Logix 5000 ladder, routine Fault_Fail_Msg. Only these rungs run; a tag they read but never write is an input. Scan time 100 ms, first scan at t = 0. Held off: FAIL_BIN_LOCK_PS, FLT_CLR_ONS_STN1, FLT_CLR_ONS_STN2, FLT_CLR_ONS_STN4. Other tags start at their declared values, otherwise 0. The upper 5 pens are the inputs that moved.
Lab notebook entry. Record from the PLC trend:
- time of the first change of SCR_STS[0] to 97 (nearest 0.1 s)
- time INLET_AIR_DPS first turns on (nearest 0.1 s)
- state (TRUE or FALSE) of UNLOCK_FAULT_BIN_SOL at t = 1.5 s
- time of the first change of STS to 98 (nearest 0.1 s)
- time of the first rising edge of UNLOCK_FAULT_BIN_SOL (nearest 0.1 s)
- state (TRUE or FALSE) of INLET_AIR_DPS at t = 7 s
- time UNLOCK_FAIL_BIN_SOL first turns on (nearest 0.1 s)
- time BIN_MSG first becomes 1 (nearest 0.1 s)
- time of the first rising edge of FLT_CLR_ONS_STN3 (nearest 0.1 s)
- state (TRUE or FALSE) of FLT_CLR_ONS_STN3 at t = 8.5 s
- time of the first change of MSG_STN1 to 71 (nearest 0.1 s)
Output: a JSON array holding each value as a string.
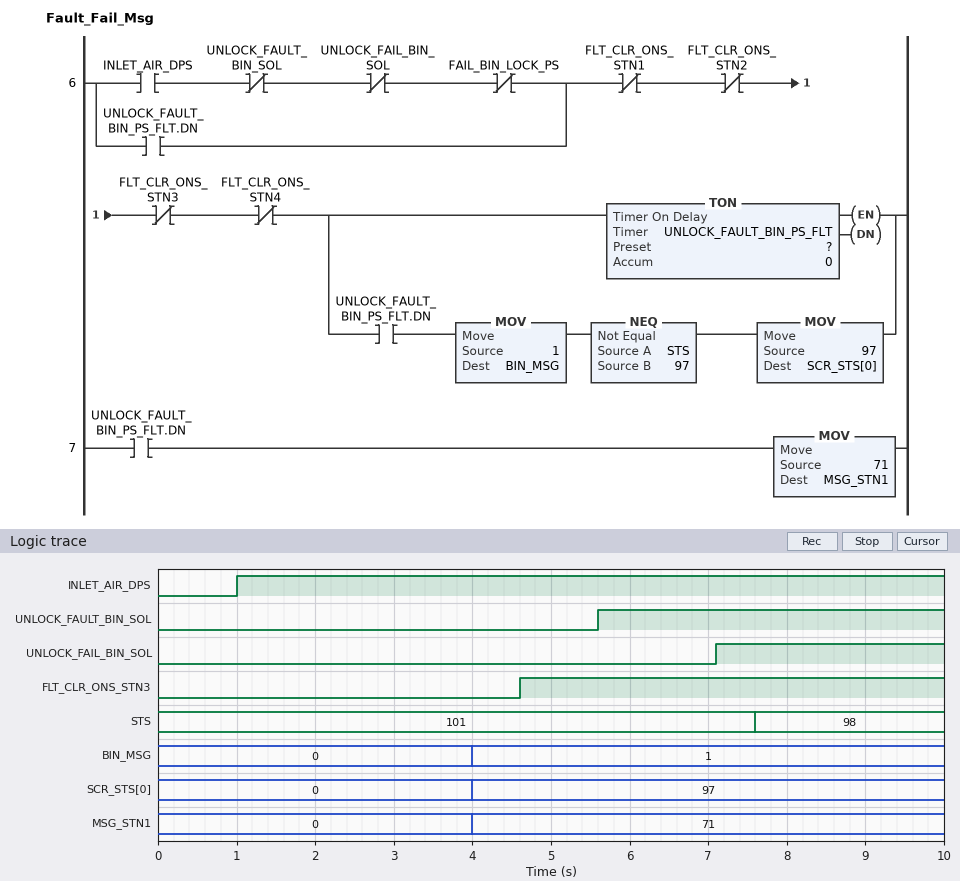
["4.0 s", "1.0 s", "FALSE", "7.6 s", "5.6 s", "TRUE", "7.1 s", "4.0 s", "4.6 s", "TRUE", "4.0 s"]
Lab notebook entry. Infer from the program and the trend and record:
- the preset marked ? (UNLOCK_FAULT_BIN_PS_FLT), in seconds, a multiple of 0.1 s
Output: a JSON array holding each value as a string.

["3.0 s"]
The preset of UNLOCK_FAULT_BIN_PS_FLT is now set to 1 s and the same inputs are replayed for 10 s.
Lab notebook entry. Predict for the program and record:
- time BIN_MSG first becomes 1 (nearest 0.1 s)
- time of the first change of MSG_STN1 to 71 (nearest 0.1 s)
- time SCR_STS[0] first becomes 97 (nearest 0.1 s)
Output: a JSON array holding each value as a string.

["2.0 s", "2.0 s", "2.0 s"]
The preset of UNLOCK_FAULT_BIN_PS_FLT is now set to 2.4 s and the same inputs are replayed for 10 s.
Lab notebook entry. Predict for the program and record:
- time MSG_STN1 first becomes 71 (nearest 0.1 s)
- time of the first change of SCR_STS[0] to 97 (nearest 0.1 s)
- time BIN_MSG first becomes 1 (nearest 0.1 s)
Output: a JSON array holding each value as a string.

["3.4 s", "3.4 s", "3.4 s"]
